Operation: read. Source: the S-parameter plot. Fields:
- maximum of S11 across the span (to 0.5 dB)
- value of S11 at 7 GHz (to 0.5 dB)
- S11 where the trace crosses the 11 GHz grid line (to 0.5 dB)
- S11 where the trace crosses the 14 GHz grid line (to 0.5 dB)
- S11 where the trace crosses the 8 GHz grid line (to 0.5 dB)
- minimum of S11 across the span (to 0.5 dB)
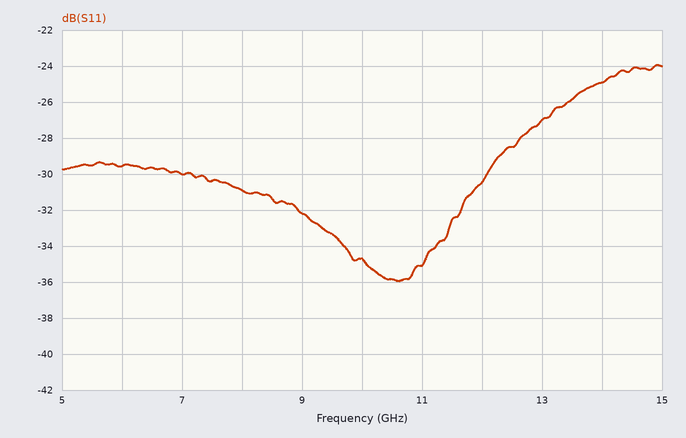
-24.0 dB
-30.0 dB
-35.0 dB
-25.0 dB
-31.0 dB
-36.0 dB
